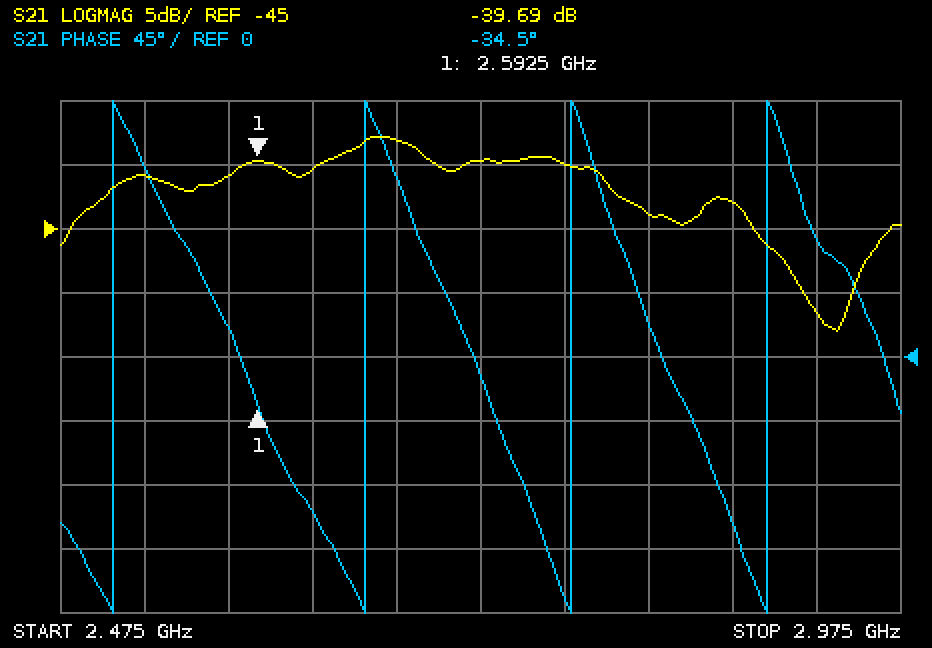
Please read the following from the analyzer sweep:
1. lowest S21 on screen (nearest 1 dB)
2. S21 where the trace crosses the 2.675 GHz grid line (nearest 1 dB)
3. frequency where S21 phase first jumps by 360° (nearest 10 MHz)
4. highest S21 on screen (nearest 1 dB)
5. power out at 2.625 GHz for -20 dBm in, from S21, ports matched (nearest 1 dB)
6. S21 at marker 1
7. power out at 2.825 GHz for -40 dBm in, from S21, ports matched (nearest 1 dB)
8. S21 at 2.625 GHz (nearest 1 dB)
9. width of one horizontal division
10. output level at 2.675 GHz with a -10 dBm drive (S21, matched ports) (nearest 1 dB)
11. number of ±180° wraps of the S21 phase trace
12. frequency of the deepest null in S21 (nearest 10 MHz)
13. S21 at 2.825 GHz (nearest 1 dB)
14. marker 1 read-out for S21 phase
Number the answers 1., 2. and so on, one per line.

1. -53 dB
2. -38 dB
3. 2.51 GHz
4. -38 dB
5. -60 dBm
6. -39.69 dB
7. -84 dBm
8. -40 dB
9. 50 MHz
10. -48 dBm
11. 4
12. 2.94 GHz
13. -44 dB
14. -34.5°
